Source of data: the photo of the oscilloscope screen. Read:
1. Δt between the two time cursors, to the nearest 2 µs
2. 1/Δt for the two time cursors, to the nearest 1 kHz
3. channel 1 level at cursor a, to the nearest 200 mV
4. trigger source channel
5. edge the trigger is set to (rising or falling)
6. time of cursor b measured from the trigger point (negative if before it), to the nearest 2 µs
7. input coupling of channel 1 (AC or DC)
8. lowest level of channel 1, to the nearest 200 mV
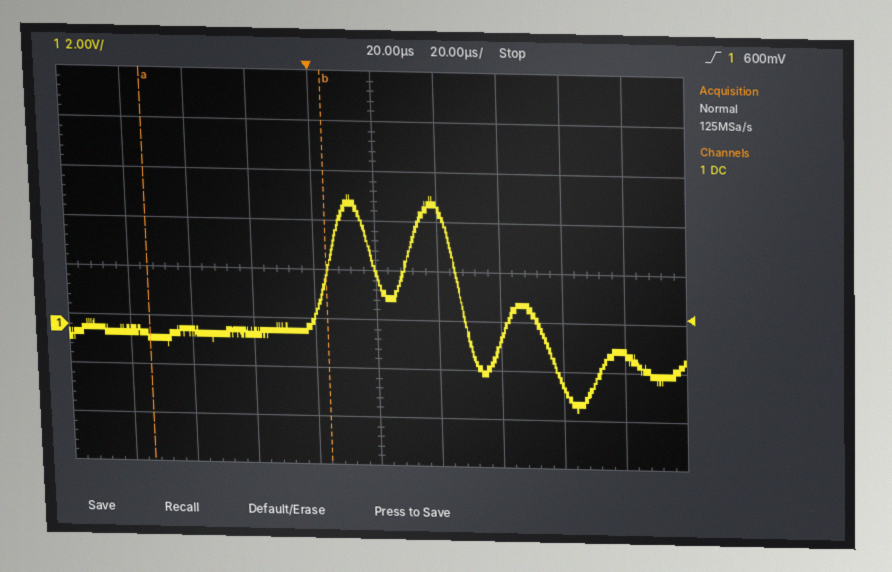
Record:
58 µs
17 kHz
-400 mV
channel 1
rising
+4 µs
DC
-3.2 V
